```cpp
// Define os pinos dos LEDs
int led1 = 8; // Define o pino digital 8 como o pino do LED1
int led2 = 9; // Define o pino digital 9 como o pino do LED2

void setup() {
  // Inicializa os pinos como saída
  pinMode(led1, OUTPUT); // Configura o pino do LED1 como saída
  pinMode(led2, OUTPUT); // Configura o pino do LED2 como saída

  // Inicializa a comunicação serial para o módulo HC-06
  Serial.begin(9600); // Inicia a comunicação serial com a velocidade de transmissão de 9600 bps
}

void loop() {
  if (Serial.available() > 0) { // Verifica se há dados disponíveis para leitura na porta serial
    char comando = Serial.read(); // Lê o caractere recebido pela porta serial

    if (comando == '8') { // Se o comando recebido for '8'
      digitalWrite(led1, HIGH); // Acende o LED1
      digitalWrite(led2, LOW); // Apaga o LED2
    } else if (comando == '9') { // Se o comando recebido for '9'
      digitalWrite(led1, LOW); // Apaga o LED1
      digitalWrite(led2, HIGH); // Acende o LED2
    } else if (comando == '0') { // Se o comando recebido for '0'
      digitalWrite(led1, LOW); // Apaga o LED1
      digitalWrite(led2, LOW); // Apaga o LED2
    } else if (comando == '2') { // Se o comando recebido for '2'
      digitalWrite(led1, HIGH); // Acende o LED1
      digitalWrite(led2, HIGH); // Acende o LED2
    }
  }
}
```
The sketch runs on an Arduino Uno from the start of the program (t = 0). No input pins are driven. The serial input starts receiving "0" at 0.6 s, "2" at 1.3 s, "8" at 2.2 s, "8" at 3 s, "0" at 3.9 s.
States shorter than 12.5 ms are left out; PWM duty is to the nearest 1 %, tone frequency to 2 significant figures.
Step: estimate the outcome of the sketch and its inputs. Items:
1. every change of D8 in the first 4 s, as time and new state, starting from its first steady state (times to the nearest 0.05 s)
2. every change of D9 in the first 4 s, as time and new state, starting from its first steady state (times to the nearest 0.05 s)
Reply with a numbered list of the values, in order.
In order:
1. 0 s low; 1.3 s high; 3.9 s low
2. 0 s low; 1.3 s high; 2.2 s low
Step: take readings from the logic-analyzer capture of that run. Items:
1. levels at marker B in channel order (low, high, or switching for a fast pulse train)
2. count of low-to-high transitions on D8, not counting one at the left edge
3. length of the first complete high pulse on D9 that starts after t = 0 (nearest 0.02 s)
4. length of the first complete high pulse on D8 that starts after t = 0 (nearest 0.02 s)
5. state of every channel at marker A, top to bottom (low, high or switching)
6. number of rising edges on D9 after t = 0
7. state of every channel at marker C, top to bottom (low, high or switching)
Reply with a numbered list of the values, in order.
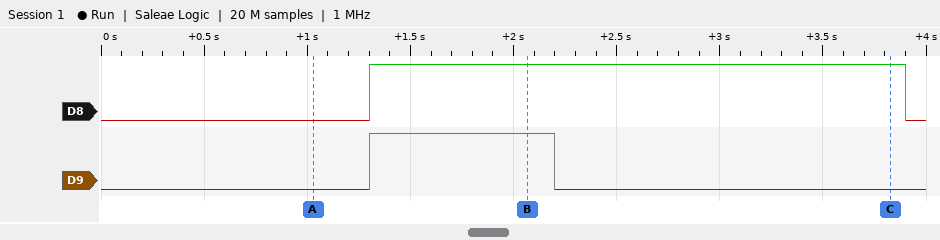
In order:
1. D8 high, D9 high
2. 1
3. 0.90 s
4. 2.60 s
5. D8 low, D9 low
6. 1
7. D8 high, D9 low
